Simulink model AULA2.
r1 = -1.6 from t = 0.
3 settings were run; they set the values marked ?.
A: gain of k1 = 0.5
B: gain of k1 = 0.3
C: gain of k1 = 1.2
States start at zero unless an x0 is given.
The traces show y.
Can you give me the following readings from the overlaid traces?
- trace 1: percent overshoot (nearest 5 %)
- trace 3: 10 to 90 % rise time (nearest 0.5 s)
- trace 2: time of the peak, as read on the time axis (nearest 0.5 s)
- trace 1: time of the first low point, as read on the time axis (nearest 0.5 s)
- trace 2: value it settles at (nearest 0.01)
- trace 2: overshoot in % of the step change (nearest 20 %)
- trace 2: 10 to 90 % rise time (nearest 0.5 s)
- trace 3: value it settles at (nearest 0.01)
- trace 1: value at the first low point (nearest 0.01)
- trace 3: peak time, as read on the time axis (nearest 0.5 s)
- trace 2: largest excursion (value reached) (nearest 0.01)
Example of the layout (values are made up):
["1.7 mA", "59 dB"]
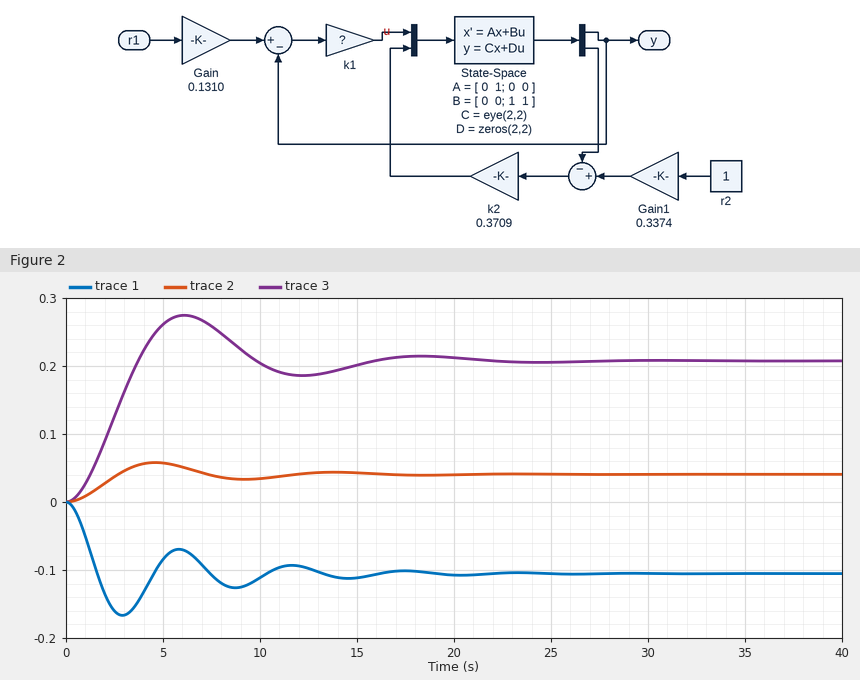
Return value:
["60 %", "2.5 s", "4.5 s", "3.0 s", "0.04", "40 %", "2.0 s", "0.21", "-0.17", "6.0 s", "0.06"]
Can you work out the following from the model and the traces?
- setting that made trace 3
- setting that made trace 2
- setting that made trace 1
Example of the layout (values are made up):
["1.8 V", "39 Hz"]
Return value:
["B", "A", "C"]
